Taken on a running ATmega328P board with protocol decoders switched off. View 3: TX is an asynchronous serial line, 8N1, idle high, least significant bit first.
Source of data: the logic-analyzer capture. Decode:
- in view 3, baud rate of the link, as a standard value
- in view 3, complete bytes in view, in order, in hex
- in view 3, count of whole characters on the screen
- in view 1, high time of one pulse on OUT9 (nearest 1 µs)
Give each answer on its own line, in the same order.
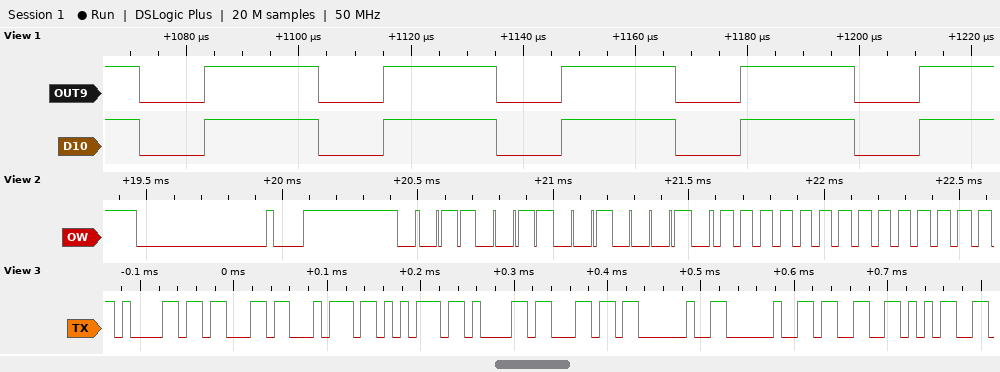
115200 baud
61 63 74 75 61 6C 20 20 33 35
10
20 µs
